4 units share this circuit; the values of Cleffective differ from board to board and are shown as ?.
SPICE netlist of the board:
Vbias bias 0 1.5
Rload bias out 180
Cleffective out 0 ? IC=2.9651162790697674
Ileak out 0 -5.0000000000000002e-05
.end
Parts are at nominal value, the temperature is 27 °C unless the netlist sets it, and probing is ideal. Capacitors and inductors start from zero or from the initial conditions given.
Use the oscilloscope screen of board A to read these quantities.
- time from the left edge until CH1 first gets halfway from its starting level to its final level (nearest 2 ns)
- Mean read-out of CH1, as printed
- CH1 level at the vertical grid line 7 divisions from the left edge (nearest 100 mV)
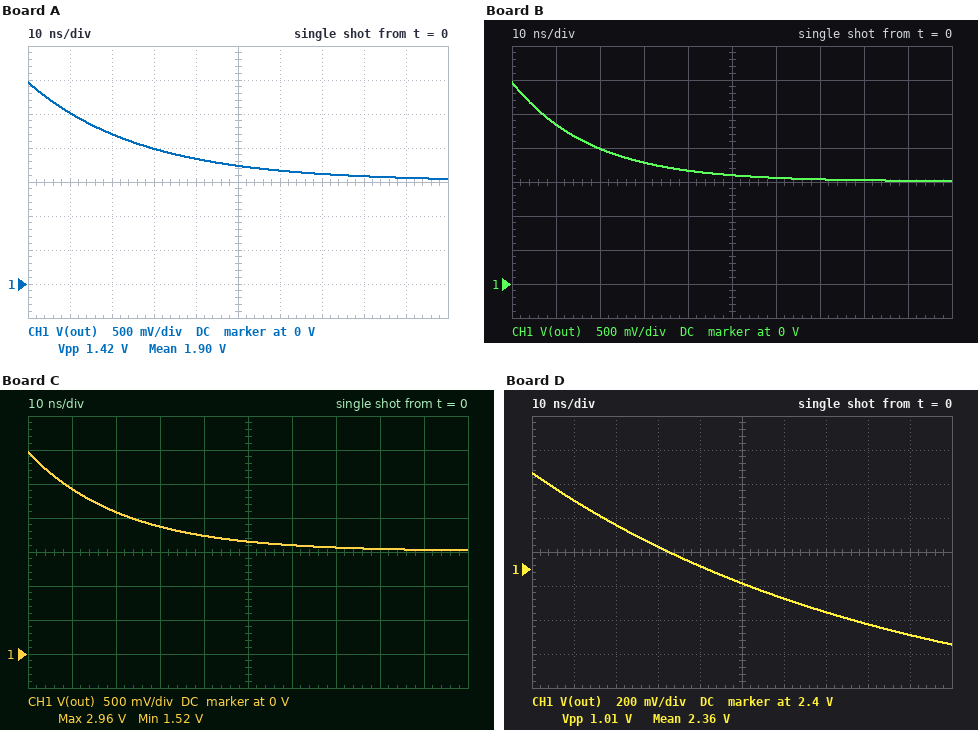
18 ns
1.90 V
1.6 V
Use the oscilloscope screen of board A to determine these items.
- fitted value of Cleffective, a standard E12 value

150 pF
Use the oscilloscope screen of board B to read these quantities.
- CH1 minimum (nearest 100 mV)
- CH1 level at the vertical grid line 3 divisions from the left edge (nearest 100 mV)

1.5 V
1.8 V
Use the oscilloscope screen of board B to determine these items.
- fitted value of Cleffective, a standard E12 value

100 pF
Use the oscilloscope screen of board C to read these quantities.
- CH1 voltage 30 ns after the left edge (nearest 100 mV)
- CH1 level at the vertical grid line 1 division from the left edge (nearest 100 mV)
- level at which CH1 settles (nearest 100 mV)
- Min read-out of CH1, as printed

1.9 V
2.4 V
1.5 V
1.52 V
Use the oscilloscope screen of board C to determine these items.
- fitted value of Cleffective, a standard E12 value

120 pF
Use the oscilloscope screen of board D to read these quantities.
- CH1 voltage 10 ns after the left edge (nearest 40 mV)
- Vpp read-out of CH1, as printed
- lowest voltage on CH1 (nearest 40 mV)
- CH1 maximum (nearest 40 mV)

2.80 V
1.01 V
1.96 V
2.96 V
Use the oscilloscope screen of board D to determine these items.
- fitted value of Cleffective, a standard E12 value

470 pF
